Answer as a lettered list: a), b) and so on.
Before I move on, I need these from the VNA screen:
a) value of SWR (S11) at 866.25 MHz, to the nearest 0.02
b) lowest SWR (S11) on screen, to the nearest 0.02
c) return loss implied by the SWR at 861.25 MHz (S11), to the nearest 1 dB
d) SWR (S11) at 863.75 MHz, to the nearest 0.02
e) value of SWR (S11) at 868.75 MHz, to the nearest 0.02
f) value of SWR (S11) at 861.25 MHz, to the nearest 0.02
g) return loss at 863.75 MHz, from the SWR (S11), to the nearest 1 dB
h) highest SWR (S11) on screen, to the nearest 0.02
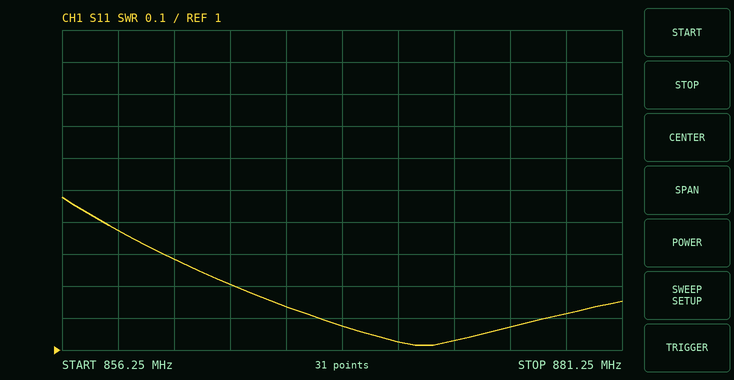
a) 1.14
b) 1.02
c) 18 dB
d) 1.20
e) 1.08
f) 1.28
g) 21 dB
h) 1.48
